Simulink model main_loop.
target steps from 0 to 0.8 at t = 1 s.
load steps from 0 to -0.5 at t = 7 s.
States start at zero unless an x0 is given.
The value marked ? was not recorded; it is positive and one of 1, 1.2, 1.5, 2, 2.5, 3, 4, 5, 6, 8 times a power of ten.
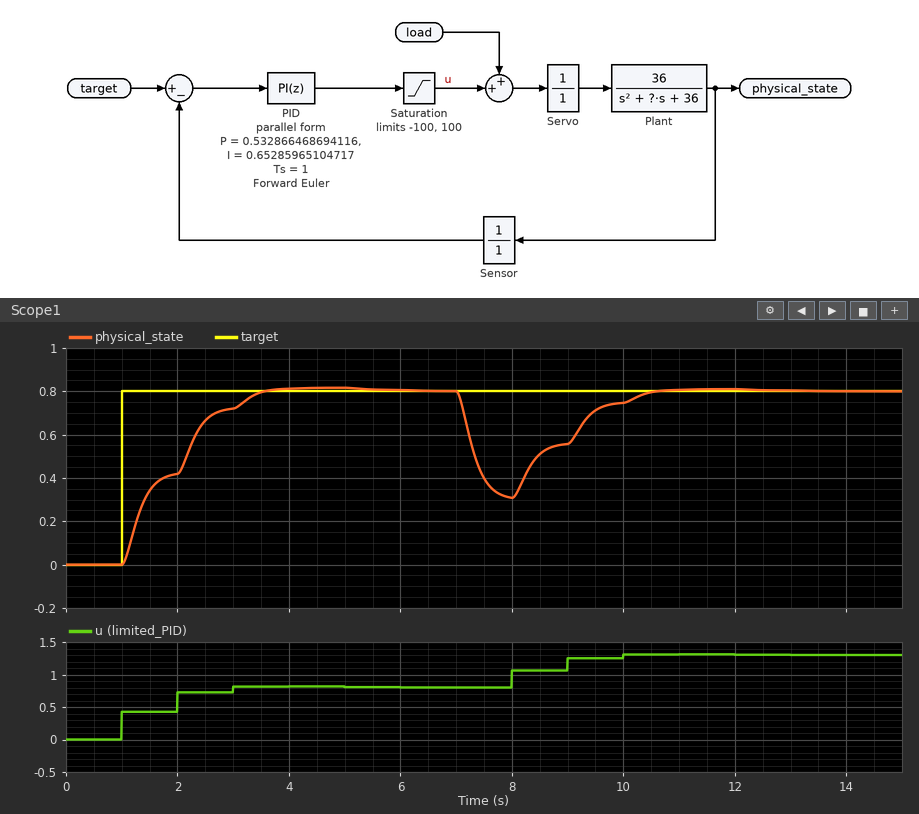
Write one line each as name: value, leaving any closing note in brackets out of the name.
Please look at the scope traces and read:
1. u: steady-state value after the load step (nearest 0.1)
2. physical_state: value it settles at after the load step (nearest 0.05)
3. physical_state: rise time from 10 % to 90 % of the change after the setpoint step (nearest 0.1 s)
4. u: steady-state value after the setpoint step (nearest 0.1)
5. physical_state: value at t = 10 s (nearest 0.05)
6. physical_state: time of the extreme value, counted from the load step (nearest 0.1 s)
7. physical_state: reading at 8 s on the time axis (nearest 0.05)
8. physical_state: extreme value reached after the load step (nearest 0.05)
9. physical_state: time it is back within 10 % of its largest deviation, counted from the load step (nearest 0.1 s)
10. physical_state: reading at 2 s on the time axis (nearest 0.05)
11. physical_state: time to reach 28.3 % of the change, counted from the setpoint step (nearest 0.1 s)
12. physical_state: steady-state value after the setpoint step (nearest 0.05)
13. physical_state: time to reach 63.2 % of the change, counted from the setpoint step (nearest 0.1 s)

u: steady-state value after the load step: 1.3
physical_state: value it settles at after the load step: 0.80
physical_state: rise time from 10 % to 90 % of the change after the setpoint step: 1.9 s
u: steady-state value after the setpoint step: 0.8
physical_state: value at t = 10 s: 0.75
physical_state: time of the extreme value, counted from the load step: 1.0 s
physical_state: reading at 8 s on the time axis: 0.30
physical_state: extreme value reached after the load step: 0.30
physical_state: time it is back within 10 % of its largest deviation, counted from the load step: 3.1 s
physical_state: reading at 2 s on the time axis: 0.40
physical_state: time to reach 28.3 % of the change, counted from the setpoint step: 0.3 s
physical_state: steady-state value after the setpoint step: 0.80
physical_state: time to reach 63.2 % of the change, counted from the setpoint step: 1.2 s
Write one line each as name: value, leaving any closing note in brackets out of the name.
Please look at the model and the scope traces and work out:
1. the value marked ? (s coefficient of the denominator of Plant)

the value marked ?: 12
